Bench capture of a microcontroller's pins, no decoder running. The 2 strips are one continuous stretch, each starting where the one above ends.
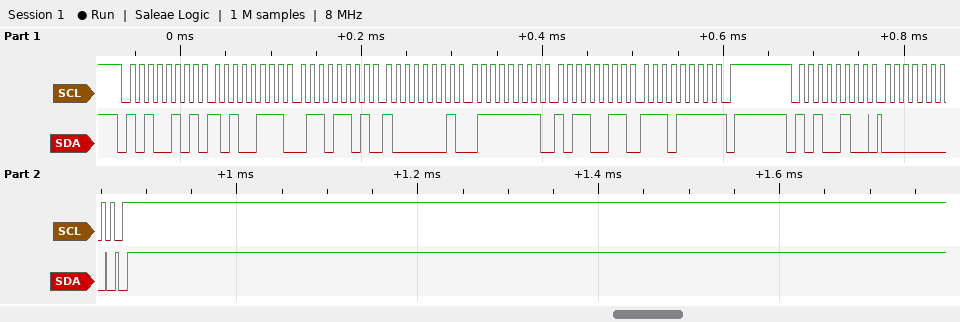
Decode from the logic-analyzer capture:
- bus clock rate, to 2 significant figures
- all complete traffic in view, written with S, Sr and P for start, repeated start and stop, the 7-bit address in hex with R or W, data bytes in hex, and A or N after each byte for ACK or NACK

100 kHz
S 52R A A7 A 6D A 81 A 7F A B3 A EF N P S 52W A 00 A P
